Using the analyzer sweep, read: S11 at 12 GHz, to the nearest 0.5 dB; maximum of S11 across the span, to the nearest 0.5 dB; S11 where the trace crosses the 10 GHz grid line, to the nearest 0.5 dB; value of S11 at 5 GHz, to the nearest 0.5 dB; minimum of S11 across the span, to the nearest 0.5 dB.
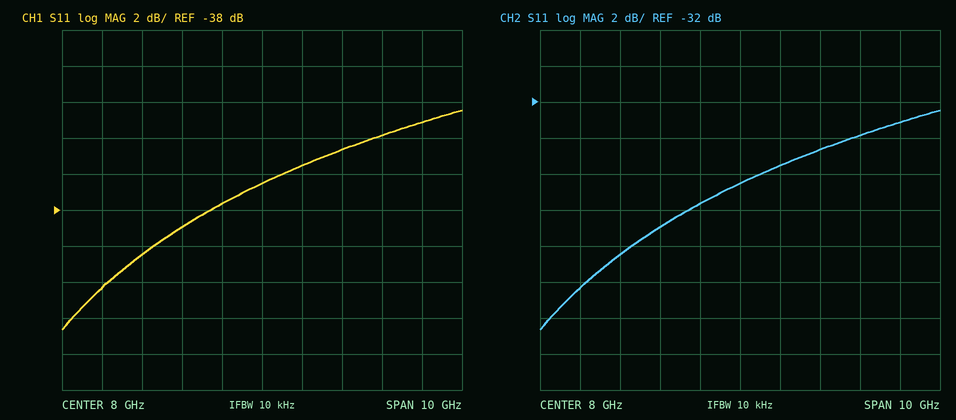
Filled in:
-33.0 dB
-32.5 dB
-34.5 dB
-40.5 dB
-44.5 dB
